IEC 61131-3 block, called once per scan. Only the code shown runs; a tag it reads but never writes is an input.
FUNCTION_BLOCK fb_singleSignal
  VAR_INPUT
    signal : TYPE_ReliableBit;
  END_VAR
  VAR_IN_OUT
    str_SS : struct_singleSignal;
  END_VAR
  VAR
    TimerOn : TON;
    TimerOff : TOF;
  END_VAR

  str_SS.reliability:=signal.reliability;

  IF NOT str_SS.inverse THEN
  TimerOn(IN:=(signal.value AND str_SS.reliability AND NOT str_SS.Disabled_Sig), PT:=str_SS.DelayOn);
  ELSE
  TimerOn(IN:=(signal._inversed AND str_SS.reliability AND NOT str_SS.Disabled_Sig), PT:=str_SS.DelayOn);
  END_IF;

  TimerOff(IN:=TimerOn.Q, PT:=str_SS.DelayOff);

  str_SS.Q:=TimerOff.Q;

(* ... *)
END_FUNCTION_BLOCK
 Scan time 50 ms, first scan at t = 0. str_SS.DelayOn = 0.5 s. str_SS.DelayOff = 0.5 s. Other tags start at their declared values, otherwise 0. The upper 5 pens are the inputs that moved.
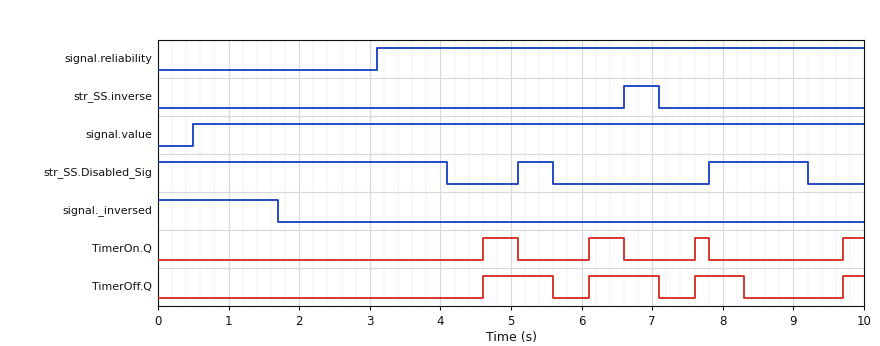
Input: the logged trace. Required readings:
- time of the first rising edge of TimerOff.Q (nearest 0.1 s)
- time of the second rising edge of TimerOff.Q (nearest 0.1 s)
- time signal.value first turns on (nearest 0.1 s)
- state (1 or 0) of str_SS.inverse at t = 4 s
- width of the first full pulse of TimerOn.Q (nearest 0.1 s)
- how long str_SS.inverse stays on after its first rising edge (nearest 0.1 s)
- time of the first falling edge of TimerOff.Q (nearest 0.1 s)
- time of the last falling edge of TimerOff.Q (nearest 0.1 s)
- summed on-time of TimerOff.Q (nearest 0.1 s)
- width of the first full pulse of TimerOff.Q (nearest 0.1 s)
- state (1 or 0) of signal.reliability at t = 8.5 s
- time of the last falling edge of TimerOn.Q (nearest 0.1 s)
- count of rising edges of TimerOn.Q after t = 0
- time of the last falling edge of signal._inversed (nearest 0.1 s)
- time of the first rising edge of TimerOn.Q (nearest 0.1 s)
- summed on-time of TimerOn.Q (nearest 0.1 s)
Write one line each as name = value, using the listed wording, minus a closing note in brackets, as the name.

time of the first rising edge of TimerOff.Q = 4.6 s
time of the second rising edge of TimerOff.Q = 6.1 s
time signal.value first turns on = 0.5 s
state (1 or 0) of str_SS.inverse at t = 4 s = 0
width of the first full pulse of TimerOn.Q = 0.5 s
how long str_SS.inverse stays on after its first rising edge = 0.5 s
time of the first falling edge of TimerOff.Q = 5.6 s
time of the last falling edge of TimerOff.Q = 8.3 s
summed on-time of TimerOff.Q = 3.0 s
width of the first full pulse of TimerOff.Q = 1.0 s
state (1 or 0) of signal.reliability at t = 8.5 s = 1
time of the last falling edge of TimerOn.Q = 7.8 s
count of rising edges of TimerOn.Q after t = 0 = 4
time of the last falling edge of signal._inversed = 1.7 s
time of the first rising edge of TimerOn.Q = 4.6 s
summed on-time of TimerOn.Q = 1.5 s
